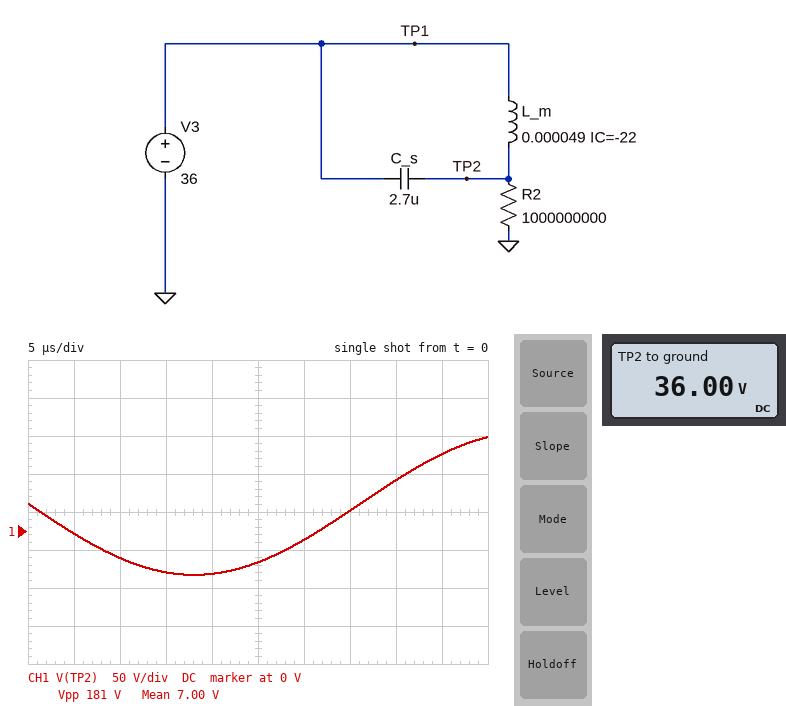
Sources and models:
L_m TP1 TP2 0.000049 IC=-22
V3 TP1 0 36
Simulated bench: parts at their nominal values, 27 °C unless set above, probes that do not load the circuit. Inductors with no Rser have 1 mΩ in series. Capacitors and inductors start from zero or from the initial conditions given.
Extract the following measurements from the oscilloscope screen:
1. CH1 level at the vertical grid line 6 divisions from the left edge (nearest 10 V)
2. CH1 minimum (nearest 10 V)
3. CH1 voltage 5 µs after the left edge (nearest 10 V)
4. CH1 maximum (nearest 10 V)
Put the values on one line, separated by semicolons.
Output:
-10 V; -60 V; 0 V; 120 V
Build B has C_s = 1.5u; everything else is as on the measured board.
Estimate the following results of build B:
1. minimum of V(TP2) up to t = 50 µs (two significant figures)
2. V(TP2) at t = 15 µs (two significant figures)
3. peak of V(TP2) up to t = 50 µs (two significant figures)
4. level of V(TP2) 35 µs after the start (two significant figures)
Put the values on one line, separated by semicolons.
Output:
-90 V; -88 V; 160 V; 140 V
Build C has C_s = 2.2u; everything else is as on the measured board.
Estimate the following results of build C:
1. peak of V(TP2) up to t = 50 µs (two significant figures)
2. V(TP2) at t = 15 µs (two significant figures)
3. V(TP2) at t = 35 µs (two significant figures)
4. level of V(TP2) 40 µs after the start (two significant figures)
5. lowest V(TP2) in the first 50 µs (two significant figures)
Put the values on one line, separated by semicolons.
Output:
140 V; -67 V; 60 V; 100 V; -68 V
